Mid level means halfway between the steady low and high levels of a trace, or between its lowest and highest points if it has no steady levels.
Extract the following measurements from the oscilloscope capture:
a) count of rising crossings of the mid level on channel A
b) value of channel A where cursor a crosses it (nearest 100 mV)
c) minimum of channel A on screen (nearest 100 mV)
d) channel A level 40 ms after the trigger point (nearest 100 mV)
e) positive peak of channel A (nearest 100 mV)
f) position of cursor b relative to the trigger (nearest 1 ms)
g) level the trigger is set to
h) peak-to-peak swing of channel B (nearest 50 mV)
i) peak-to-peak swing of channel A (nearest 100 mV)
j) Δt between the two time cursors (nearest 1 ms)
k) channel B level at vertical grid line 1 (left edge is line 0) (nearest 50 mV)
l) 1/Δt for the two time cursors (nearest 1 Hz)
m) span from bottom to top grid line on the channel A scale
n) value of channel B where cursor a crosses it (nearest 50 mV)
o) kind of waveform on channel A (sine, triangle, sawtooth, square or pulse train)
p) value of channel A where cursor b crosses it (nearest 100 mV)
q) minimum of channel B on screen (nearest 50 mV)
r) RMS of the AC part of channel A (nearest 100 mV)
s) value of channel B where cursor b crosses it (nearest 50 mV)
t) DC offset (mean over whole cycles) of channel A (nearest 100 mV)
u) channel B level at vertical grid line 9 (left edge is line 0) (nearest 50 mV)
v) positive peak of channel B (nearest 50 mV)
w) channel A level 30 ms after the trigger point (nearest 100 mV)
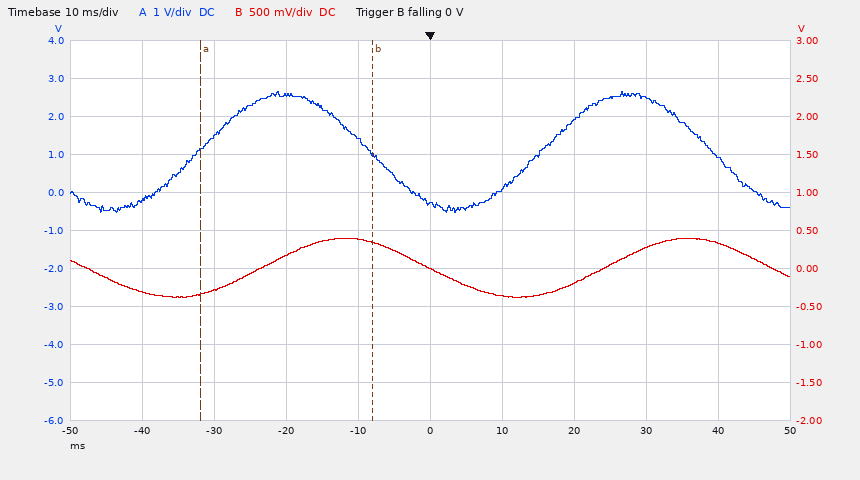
2
1.1 V
-500 mV
900 mV
2.7 V
-8 ms
0 V
800 mV
3.2 V
24 ms
-300 mV
42 Hz
10 V
-350 mV
sine
1.0 V
-400 mV
1.1 V
350 mV
1.1 V
350 mV
400 mV
2.5 V
